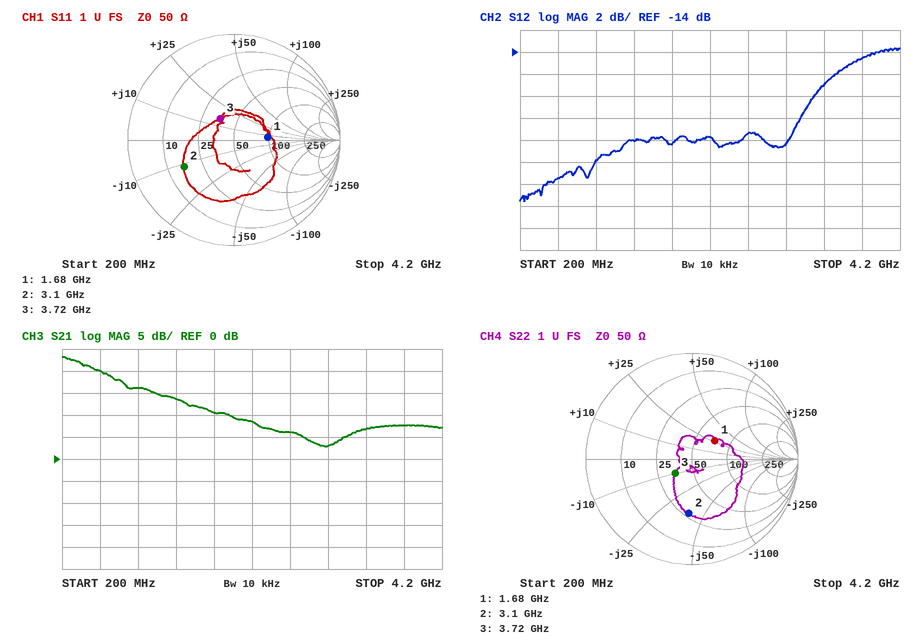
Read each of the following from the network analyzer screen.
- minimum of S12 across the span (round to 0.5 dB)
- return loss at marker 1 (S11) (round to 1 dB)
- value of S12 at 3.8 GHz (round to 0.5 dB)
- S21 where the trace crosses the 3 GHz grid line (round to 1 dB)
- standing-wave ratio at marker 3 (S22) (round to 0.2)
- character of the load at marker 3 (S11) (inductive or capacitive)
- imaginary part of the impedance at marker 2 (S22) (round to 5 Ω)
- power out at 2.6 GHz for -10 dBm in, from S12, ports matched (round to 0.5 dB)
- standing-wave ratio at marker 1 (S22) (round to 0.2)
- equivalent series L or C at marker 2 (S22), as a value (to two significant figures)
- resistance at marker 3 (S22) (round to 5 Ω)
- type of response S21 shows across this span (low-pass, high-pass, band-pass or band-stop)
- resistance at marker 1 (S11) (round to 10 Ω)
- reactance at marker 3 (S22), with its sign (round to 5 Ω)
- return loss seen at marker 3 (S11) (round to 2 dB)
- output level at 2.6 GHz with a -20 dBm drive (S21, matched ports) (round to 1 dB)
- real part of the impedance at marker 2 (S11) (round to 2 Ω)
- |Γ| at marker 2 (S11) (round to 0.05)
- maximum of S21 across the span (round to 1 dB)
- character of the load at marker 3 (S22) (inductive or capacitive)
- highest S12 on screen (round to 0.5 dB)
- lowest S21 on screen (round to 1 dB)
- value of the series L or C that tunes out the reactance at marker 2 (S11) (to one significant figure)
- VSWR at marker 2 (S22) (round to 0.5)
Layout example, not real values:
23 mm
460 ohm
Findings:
-27.5 dB
10 dB
-14.5 dB
3 dB
1.6
inductive
-40 Ω
-31.5 dBm
1.8
1.3 pF
35 Ω
low-pass
100 Ω
-10 Ω
12 dB
-14 dBm
16 Ω
0.55
23 dB
capacitive
-13.5 dB
3 dB
600 pH
3.0
